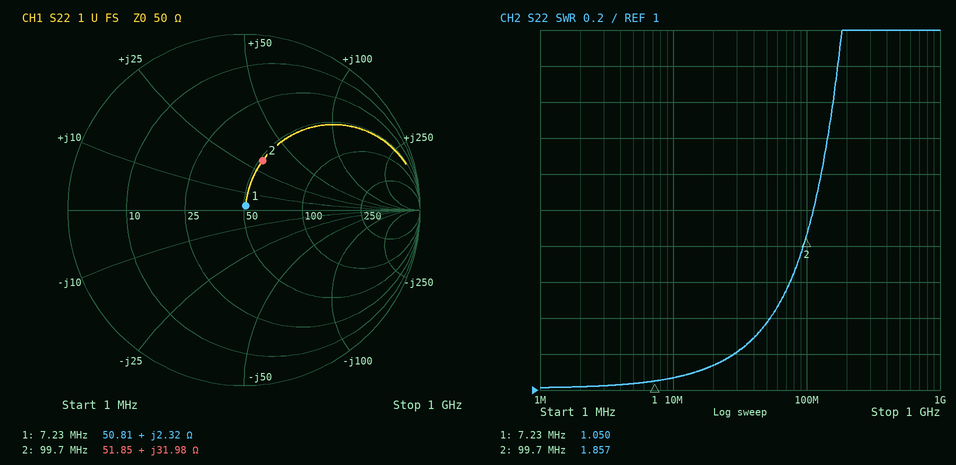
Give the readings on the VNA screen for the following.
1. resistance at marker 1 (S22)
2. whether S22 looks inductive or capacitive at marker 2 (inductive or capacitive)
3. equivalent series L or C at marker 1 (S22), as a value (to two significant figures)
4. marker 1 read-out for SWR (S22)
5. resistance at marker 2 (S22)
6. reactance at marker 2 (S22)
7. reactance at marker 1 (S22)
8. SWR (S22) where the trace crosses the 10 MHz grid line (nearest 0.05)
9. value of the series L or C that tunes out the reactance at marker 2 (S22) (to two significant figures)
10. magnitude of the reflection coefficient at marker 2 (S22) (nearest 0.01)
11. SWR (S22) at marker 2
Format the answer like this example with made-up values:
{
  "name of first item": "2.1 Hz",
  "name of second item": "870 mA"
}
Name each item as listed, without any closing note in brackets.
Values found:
{
  "resistance at marker 1": "50.81 Ω",
  "whether S22 looks inductive or capacitive at marker 2": "inductive",
  "equivalent series L or C at marker 1 (S22), as a value": "51 nH",
  "marker 1 read-out for SWR": "1.050",
  "resistance at marker 2": "51.85 Ω",
  "reactance at marker 2": "+31.98 Ω",
  "reactance at marker 1": "+2.32 Ω",
  "SWR (S22) where the trace crosses the 10 MHz grid line": "1.05",
  "value of the series L or C that tunes out the reactance at marker 2 (S22)": "50 pF",
  "magnitude of the reflection coefficient at marker 2 (S22)": "0.30",
  "SWR (S22) at marker 2": "1.857"
}
